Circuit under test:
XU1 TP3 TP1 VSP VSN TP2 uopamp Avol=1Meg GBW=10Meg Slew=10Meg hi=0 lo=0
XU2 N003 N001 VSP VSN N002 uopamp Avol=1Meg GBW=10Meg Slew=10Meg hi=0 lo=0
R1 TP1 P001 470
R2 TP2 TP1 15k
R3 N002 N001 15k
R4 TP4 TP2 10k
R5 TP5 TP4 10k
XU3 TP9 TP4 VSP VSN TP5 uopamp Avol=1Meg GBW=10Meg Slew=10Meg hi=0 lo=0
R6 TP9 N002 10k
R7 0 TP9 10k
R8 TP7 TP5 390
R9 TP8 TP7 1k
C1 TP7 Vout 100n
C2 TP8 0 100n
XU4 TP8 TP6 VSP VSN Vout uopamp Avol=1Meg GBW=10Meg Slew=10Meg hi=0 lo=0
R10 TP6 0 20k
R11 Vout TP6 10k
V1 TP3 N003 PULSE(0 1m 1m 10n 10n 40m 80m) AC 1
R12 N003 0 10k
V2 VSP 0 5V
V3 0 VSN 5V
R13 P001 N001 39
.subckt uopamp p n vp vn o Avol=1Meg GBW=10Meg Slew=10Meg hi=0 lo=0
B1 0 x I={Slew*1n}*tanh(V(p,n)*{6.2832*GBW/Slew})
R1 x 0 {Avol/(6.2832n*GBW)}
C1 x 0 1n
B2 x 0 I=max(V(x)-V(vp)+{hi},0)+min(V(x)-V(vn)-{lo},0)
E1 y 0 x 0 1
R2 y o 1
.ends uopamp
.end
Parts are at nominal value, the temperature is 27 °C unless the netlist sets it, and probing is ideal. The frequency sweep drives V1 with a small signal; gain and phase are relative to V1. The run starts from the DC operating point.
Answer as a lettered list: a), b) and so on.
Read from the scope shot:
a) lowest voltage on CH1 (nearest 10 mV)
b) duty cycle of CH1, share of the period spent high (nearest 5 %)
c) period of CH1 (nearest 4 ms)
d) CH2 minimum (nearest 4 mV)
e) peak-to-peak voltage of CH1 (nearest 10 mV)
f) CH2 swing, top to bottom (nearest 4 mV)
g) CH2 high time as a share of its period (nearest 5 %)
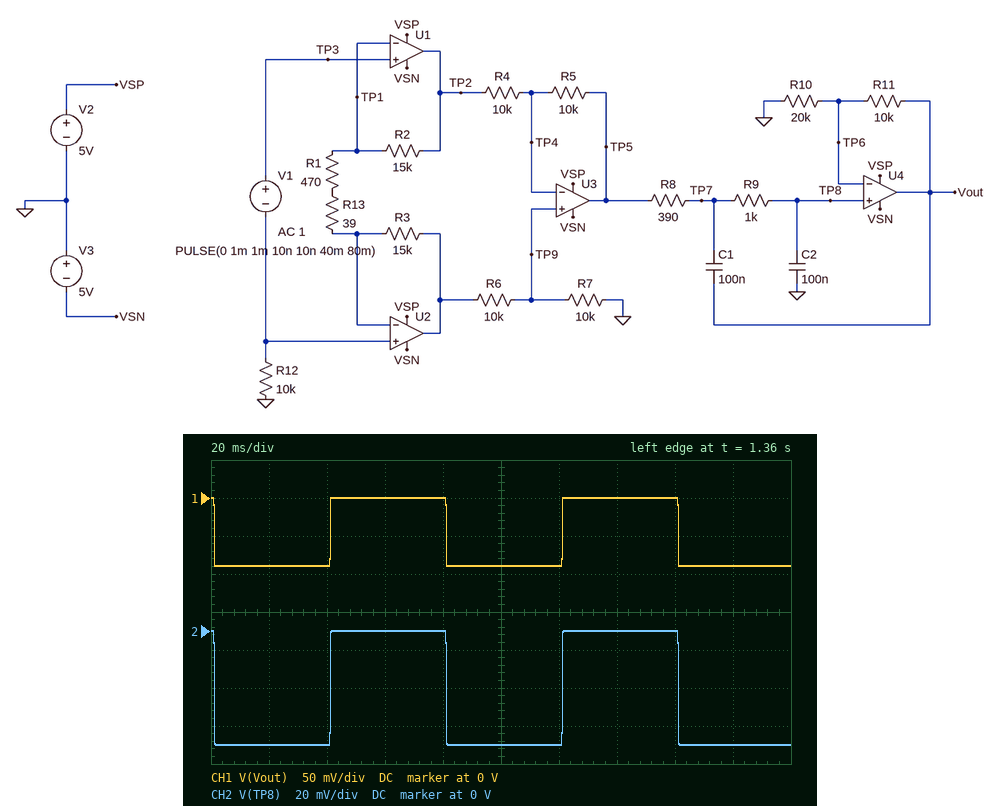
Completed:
a) -90 mV
b) 50 %
c) 80 ms
d) -60 mV
e) 90 mV
f) 60 mV
g) 50 %
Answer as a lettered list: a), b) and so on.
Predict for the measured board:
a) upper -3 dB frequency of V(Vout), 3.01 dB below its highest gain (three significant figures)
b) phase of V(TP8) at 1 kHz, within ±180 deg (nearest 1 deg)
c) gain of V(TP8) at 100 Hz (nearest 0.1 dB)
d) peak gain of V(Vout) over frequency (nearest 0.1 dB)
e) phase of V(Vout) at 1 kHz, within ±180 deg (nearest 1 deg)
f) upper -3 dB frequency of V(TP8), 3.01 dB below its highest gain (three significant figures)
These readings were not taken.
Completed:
a) 1.75 kHz
b) 138 deg
c) 35.5 dB
d) 39.1 dB
e) 138 deg
f) 1.75 kHz
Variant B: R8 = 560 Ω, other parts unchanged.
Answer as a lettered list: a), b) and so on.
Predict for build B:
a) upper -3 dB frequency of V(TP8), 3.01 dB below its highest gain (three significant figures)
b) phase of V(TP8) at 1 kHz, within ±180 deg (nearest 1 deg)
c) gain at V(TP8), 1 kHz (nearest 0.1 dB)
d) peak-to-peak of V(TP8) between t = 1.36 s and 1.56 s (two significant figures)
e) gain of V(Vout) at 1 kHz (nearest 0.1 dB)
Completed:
a) 1.70 kHz
b) 134 deg
c) 34.6 dB
d) 61 mV
e) 38.1 dB
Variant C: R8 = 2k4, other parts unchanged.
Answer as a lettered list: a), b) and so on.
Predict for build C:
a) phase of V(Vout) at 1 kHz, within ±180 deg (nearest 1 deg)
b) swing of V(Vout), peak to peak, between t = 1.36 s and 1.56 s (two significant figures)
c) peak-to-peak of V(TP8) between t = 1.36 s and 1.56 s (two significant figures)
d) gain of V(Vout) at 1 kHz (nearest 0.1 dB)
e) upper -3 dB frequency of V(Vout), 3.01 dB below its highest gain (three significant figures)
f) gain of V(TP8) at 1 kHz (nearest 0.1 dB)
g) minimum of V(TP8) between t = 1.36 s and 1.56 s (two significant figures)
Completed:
a) 92 deg
b) 99 mV
c) 66 mV
d) 36.3 dB
e) 1.02 kHz
f) 32.7 dB
g) -63 mV
